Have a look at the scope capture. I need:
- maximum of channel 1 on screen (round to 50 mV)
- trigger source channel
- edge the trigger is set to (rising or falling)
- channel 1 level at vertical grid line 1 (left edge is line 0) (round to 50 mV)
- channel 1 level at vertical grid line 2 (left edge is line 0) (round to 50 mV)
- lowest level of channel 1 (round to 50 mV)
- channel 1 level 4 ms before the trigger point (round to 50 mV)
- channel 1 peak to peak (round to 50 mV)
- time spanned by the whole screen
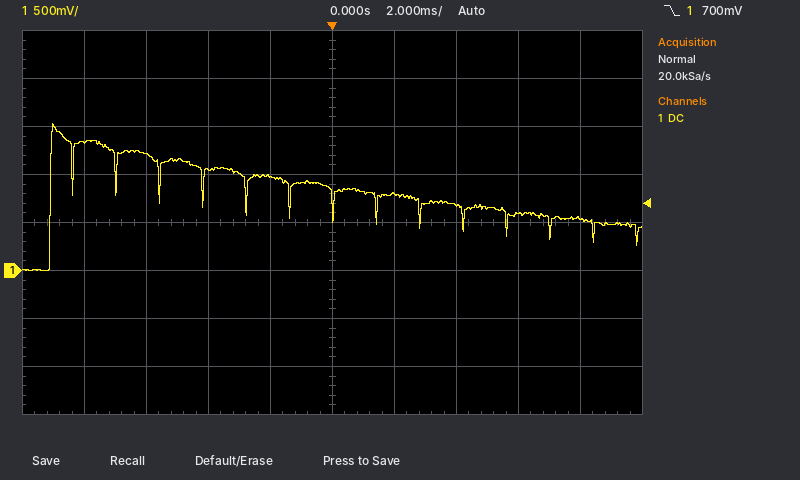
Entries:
1.55 V
channel 1
falling
1.35 V
1.20 V
0 mV
1.05 V
1.55 V
20 ms
